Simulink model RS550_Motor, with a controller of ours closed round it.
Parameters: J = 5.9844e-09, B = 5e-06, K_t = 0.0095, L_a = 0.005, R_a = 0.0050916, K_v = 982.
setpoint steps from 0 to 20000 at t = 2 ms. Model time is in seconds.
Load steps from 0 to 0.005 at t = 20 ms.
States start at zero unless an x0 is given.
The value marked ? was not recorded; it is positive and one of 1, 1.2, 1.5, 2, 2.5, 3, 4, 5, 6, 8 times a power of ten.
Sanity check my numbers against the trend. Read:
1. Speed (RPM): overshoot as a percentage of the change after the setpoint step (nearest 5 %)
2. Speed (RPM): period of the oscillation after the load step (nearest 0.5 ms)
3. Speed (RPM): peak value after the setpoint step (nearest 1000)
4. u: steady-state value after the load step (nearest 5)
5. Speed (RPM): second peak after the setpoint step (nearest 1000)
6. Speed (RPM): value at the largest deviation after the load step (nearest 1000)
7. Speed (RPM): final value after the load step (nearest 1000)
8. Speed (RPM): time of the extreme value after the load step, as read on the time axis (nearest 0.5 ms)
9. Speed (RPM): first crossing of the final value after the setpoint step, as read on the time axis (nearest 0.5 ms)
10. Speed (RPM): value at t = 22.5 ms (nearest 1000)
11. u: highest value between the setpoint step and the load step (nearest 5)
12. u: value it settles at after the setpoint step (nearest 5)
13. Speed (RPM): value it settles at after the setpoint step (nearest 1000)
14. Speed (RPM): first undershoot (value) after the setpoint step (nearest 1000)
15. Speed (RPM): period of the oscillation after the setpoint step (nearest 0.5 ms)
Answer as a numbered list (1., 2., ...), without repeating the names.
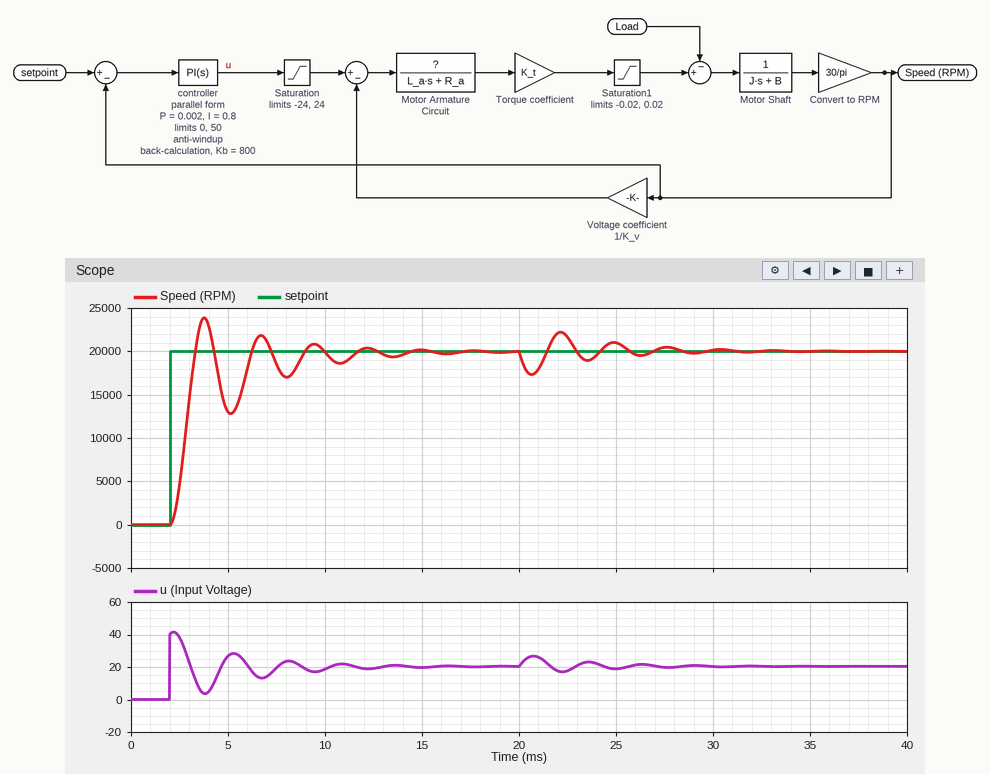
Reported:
1. 20 %
2. 3.0 ms
3. 24000
4. 20
5. 22000
6. 17000
7. 20000
8. 20.5 ms
9. 3.5 ms
10. 22000
11. 40
12. 20
13. 20000
14. 13000
15. 3.0 ms
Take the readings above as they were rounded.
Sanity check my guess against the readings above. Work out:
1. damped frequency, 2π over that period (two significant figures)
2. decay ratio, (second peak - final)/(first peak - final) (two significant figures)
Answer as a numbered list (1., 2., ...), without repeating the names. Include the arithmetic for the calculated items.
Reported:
1. 2π / 3 = 2.1 rad/ms
2. (22000 - 20000) / (24000 - 20000) = 0.50
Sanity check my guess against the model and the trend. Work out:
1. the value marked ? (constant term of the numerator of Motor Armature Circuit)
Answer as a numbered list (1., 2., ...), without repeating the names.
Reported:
1. 0.6
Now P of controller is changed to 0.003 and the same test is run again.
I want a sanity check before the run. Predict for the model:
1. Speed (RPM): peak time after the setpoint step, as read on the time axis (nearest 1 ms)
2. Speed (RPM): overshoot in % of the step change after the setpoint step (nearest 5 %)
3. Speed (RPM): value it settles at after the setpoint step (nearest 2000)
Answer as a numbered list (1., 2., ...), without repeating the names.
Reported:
1. 4 ms
2. 15 %
3. 20000
